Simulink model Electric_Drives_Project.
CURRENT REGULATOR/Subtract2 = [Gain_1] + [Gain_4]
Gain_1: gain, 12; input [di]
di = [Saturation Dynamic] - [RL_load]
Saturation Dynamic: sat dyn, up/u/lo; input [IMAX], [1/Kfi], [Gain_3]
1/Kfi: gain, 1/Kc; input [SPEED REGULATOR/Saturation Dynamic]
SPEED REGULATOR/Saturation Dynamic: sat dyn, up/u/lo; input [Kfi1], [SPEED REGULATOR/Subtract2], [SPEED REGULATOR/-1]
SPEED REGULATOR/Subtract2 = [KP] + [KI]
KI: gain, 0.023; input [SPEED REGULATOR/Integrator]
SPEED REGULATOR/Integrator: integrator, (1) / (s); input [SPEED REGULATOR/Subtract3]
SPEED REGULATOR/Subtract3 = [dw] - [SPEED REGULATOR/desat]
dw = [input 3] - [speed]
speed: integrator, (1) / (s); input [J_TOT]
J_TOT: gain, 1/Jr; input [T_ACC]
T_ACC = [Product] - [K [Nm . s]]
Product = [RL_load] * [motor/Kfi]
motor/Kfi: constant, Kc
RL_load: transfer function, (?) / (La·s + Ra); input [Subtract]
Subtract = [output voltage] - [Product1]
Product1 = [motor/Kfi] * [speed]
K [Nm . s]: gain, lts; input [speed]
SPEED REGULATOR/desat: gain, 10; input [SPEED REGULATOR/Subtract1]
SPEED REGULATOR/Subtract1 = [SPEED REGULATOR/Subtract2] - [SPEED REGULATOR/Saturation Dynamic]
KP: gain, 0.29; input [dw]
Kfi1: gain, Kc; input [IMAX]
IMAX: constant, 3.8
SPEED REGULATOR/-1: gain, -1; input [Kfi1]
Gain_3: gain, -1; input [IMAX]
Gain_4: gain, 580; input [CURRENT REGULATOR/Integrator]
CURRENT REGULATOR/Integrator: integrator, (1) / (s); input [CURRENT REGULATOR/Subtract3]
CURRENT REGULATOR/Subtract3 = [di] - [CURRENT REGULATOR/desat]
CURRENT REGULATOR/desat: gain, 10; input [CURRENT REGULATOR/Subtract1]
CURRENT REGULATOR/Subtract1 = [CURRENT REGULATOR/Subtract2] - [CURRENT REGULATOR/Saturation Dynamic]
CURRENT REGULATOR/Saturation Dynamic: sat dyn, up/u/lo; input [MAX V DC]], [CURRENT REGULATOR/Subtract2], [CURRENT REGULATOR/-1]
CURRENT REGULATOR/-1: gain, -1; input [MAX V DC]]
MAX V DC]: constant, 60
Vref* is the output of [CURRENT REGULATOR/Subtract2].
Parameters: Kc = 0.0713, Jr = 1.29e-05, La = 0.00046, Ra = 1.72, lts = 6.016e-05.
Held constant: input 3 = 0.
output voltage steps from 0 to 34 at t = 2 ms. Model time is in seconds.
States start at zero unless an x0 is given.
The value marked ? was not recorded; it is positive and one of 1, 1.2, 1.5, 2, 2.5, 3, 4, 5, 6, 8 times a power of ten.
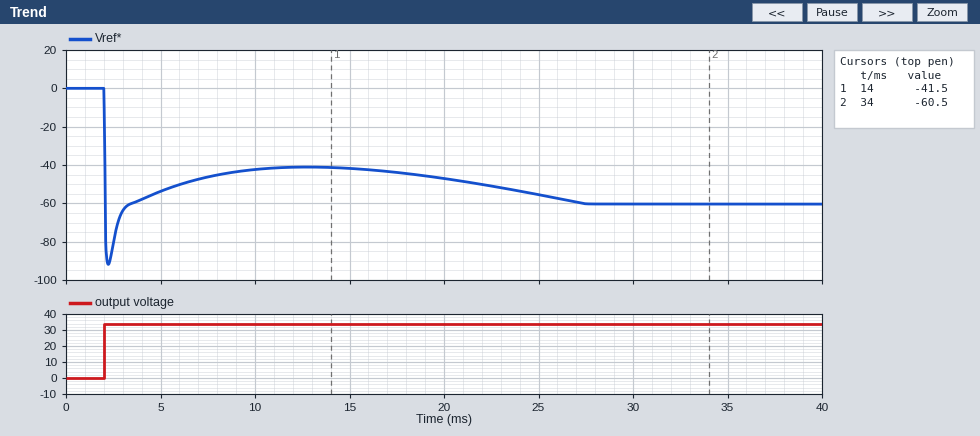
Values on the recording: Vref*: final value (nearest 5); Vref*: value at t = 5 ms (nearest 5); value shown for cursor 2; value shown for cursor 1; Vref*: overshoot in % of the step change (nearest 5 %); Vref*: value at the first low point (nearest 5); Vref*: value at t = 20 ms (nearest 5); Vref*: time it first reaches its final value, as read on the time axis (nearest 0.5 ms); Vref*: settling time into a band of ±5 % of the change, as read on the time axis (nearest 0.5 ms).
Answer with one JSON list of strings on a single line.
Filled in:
["-60", "-55", "-60.5", "-41.5", "50 %", "-90", "-45", "2.0 ms", "26.0 ms"]
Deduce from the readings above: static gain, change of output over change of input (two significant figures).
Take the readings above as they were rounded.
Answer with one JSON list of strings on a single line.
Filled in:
["-1.8"]
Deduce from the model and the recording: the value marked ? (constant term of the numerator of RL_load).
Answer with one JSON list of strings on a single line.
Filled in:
["0.5"]
